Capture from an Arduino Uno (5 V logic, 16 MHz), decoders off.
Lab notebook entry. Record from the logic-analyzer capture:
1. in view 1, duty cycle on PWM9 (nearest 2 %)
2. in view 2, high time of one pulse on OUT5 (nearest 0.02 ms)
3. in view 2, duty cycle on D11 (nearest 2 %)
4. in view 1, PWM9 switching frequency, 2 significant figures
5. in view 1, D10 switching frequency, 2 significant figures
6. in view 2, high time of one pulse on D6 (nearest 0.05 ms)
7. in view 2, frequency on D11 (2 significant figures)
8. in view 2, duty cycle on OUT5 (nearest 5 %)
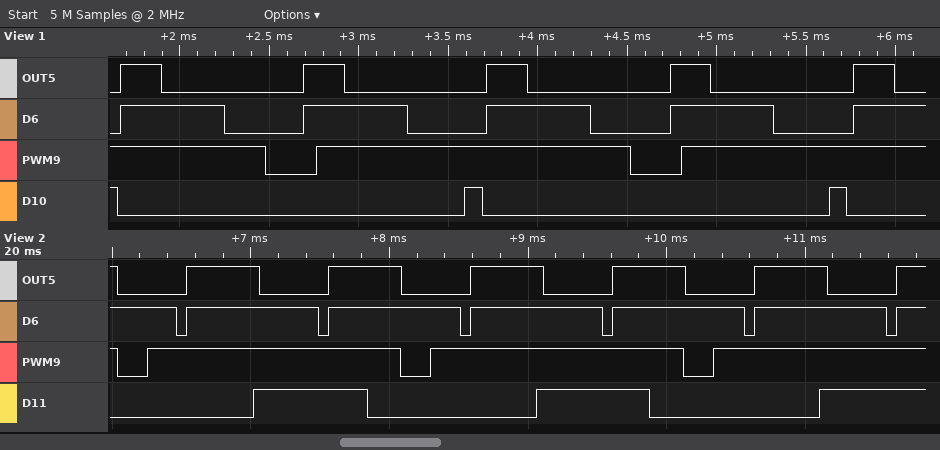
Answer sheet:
86 %
0.52 ms
40 %
490 Hz
490 Hz
0.95 ms
490 Hz
50 %
